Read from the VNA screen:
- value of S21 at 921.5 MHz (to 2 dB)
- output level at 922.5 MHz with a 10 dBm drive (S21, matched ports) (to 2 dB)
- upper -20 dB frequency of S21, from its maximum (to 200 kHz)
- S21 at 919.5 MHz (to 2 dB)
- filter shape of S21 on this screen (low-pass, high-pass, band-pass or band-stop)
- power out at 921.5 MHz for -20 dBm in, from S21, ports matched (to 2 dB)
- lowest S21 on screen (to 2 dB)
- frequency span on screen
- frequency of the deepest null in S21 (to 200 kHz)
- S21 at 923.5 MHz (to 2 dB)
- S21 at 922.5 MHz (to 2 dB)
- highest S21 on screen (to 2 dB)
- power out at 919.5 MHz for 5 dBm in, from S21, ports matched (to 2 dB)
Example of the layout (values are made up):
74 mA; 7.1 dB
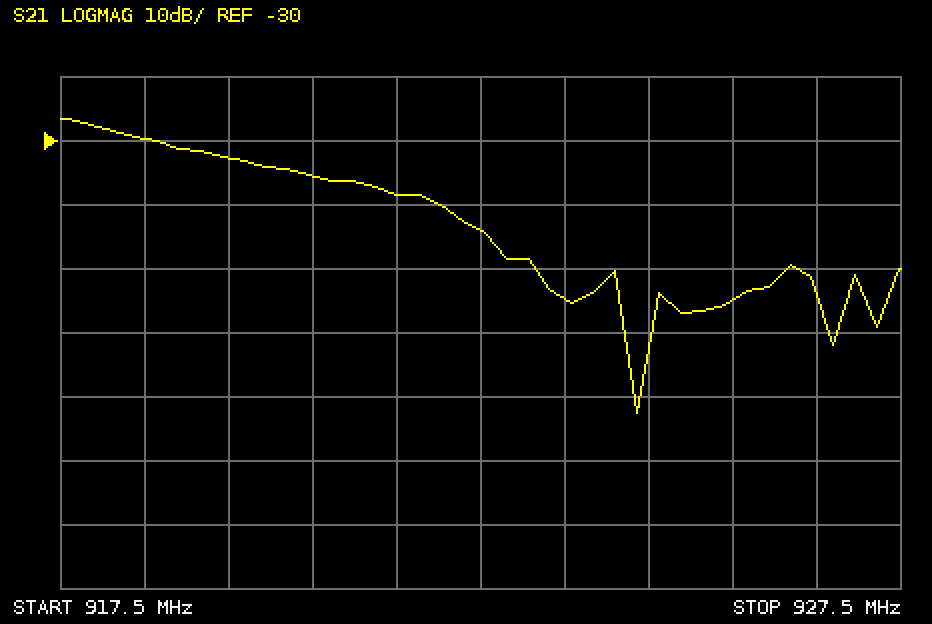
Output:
-38 dB; -34 dBm; 922.6 MHz; -32 dB; low-pass; -58 dBm; -72 dB; 10 MHz; 924.4 MHz; -54 dB; -44 dB; -26 dB; -28 dBm
